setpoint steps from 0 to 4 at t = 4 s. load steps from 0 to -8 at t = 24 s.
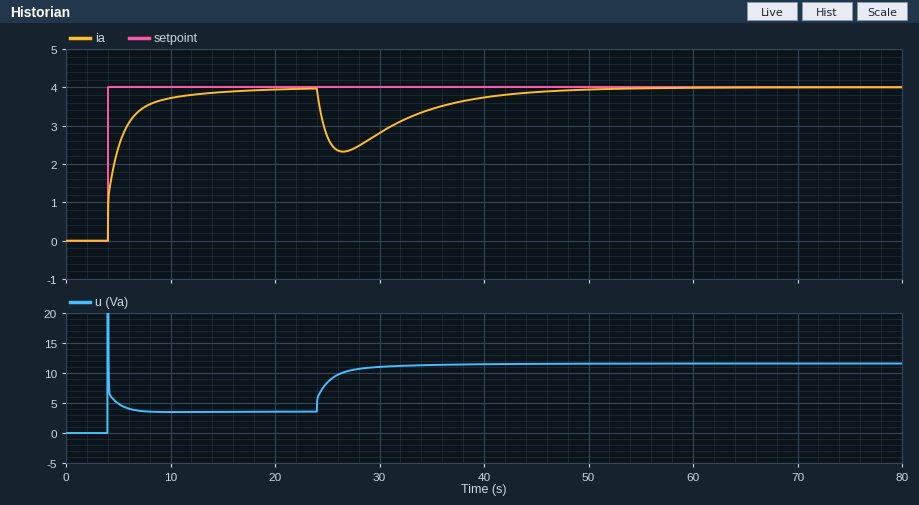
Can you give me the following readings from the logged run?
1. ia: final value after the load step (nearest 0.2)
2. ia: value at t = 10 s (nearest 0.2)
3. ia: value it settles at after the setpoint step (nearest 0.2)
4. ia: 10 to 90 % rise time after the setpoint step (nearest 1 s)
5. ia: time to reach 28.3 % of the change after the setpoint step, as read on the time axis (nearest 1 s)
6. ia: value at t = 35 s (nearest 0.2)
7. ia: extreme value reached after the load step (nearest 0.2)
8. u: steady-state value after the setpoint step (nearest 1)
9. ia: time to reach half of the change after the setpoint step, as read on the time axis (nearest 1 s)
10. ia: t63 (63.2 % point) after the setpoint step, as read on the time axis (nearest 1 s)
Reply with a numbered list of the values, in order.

1. 4.0
2. 3.8
3. 4.0
4. 4 s
5. 4 s
6. 3.4
7. 2.4
8. 4
9. 5 s
10. 5 s
